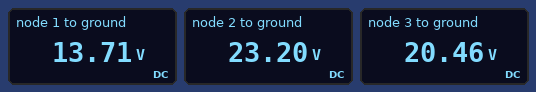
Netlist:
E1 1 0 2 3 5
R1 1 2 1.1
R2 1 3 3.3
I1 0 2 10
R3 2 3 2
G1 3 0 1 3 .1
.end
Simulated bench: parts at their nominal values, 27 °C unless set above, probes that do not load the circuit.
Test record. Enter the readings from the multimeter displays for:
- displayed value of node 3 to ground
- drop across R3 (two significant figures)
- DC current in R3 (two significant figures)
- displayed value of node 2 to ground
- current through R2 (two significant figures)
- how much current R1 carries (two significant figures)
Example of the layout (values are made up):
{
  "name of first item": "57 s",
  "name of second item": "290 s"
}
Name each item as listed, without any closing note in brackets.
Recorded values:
{
  "displayed value of node 3 to ground": "20.46 V",
  "drop across R3": "2.7 V",
  "DC current in R3": "1.4 A",
  "displayed value of node 2 to ground": "23.20 V",
  "current through R2": "2.0 A",
  "how much current R1 carries": "8.6 A"
}
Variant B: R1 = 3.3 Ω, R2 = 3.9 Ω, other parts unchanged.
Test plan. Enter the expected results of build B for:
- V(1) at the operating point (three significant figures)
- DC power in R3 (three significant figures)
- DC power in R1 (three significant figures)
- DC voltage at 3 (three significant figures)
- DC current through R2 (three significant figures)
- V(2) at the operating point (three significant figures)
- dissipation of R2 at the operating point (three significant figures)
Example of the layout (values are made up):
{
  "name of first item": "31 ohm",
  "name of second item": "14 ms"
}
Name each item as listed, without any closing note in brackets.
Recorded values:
{
  "V(1) at the operating point": "28.2 V",
  "DC power in R3": "15.9 W",
  "DC power in R1": "170 W",
  "DC voltage at 3": "46.3 V",
  "DC current through R2": "4.63 A",
  "V(2) at the operating point": "51.9 V",
  "dissipation of R2 at the operating point": "83.5 W"
}
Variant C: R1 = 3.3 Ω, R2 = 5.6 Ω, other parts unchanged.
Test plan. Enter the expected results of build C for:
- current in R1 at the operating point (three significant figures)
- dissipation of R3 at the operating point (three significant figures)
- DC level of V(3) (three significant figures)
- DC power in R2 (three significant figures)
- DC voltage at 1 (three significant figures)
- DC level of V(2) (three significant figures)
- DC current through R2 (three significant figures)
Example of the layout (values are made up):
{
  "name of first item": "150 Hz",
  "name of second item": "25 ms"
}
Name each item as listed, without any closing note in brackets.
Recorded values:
{
  "current in R1 at the operating point": "8.17 A",
  "dissipation of R3 at the operating point": "6.70 W",
  "DC level of V(3)": "41.6 V",
  "DC power in R2": "96.9 W",
  "DC voltage at 1": "18.3 V",
  "DC level of V(2)": "45.3 V",
  "DC current through R2": "4.16 A"
}
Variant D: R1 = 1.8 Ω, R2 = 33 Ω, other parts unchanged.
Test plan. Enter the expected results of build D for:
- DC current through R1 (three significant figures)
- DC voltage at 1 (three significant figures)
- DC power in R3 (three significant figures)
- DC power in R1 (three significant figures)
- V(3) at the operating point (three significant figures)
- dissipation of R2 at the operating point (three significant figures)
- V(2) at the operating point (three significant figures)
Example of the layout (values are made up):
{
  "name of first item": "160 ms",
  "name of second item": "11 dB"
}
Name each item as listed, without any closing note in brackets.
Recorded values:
{
  "DC current through R1": "11.7 A",
  "DC voltage at 1": "-17.1 V",
  "DC power in R3": "5.82 W",
  "DC power in R1": "247 W",
  "V(3) at the operating point": "7.42 V",
  "dissipation of R2 at the operating point": "18.2 W",
  "V(2) at the operating point": "4.01 V"
}
